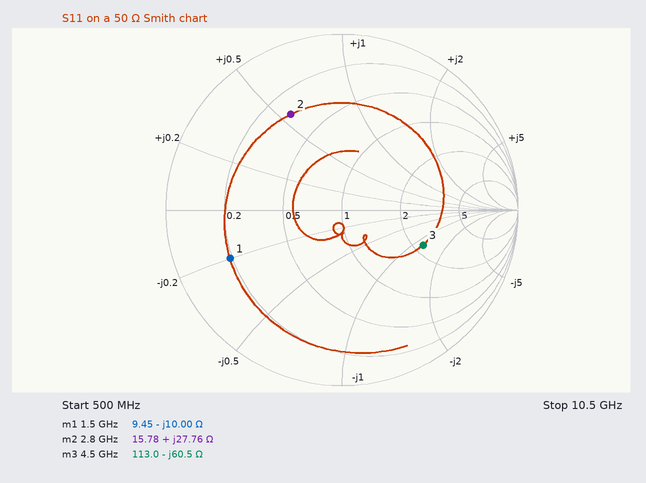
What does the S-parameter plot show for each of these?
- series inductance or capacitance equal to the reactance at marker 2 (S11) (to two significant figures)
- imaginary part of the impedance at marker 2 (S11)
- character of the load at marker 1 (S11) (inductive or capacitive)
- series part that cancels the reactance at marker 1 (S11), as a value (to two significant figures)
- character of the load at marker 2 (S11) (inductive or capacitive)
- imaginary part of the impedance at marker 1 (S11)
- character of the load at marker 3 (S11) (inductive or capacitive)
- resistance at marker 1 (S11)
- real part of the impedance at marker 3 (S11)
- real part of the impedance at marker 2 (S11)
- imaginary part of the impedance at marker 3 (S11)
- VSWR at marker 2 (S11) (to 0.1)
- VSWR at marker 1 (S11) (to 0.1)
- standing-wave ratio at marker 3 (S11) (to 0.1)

1.6 nH
+27.76 Ω
capacitive
1.1 nH
inductive
-10.00 Ω
capacitive
9.45 Ω
113.0 Ω
15.78 Ω
-60.5 Ω
4.2
5.5
3.0
